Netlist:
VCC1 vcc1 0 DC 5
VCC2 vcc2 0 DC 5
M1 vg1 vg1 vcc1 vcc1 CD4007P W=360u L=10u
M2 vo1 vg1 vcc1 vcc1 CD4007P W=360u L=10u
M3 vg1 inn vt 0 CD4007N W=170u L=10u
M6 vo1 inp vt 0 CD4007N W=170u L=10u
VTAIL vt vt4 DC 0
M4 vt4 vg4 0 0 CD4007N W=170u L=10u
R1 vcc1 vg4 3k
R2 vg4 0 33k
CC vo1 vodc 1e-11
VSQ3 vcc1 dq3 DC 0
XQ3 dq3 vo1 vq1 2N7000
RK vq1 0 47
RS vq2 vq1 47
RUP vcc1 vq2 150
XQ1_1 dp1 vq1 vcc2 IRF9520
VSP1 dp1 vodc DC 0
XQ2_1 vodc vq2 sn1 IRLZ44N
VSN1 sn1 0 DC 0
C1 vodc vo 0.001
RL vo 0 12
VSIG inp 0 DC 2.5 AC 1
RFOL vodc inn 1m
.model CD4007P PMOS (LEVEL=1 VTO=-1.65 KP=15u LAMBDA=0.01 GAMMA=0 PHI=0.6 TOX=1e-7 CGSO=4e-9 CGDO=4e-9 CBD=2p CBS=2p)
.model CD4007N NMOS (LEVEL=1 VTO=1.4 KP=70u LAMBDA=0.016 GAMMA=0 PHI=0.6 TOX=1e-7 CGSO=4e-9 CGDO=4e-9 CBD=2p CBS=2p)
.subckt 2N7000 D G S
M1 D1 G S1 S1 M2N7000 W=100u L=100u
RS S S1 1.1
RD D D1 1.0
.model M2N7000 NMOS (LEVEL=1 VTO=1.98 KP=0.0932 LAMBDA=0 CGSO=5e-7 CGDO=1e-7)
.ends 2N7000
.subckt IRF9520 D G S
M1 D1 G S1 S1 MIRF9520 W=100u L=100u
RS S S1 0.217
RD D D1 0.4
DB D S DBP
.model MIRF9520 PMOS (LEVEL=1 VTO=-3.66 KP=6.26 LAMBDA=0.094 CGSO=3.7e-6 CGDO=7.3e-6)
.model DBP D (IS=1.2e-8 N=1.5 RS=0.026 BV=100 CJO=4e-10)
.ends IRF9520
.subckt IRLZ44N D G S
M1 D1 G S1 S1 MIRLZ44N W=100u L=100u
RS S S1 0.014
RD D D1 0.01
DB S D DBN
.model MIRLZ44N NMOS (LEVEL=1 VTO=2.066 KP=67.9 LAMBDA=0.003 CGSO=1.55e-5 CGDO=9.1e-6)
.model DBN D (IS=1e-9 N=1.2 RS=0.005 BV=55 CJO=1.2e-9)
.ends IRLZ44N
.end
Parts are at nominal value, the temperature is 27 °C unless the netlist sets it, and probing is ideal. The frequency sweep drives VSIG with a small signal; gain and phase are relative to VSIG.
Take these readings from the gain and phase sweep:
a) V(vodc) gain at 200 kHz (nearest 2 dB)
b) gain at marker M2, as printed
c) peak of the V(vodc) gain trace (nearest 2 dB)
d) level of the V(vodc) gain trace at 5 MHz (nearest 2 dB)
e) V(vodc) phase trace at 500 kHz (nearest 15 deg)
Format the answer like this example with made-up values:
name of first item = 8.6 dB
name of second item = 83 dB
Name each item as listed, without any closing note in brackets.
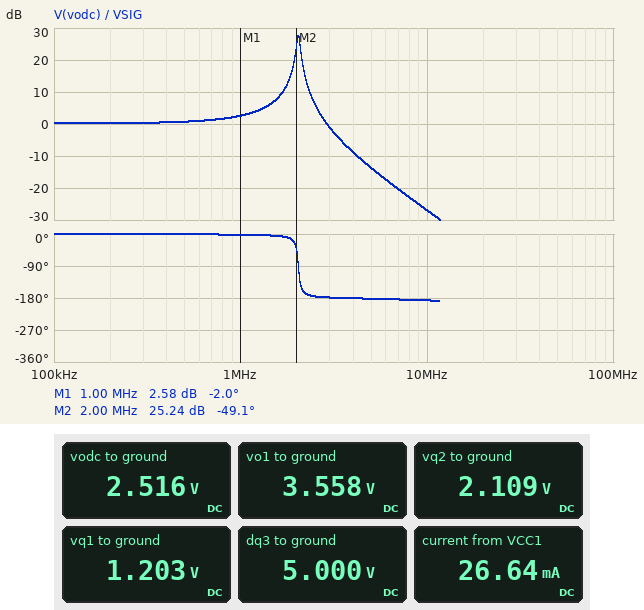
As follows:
V(vodc) gain at 200 kHz = 0 dB
gain at marker M2, as printed = 25.24 dB
peak of the V(vodc) gain trace = 28 dB
level of the V(vodc) gain trace at 5 MHz = -14 dB
V(vodc) phase trace at 500 kHz = 0 deg
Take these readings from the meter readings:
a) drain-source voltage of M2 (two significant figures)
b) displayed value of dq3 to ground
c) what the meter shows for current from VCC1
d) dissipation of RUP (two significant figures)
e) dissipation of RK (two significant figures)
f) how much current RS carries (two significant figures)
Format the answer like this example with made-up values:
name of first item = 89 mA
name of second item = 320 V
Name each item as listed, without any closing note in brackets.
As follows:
drain-source voltage of M2 = -1.4 V
displayed value of dq3 to ground = 5.000 V
what the meter shows for current from VCC1 = 26.64 mA
dissipation of RUP = 56 mW
dissipation of RK = 31 mW
how much current RS carries = 19 mA
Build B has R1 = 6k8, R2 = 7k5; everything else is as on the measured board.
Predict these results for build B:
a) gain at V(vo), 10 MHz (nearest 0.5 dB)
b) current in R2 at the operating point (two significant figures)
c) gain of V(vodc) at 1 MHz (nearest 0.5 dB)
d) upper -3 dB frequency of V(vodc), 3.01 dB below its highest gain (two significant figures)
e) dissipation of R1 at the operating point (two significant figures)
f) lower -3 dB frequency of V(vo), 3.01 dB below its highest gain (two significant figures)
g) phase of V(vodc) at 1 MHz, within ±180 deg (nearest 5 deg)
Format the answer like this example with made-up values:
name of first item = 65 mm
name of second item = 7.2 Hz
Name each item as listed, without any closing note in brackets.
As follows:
gain at V(vo), 10 MHz = -30.5 dB
current in R2 at the operating point = 350 µA
gain of V(vodc) at 1 MHz = 3.5 dB
upper -3 dB frequency of V(vodc), 3.01 dB below its highest gain = 1.8 MHz
dissipation of R1 at the operating point = 830 µW
lower -3 dB frequency of V(vo), 3.01 dB below its highest gain = 1.7 MHz
phase of V(vodc) at 1 MHz, within ±180 deg = -5 deg
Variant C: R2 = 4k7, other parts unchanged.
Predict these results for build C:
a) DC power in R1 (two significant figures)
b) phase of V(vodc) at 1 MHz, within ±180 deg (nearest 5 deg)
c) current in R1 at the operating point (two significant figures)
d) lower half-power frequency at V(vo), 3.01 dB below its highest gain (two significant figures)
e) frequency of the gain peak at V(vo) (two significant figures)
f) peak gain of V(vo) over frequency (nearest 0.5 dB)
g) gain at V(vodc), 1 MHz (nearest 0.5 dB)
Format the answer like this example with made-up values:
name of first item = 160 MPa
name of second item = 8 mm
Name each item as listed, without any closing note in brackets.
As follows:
DC power in R1 = 1.3 mW
phase of V(vodc) at 1 MHz, within ±180 deg = -5 deg
current in R1 at the operating point = 650 µA
lower half-power frequency at V(vo), 3.01 dB below its highest gain = 1.8 MHz
frequency of the gain peak at V(vo) = 1.9 MHz
peak gain of V(vo) over frequency = 25.5 dB
gain at V(vodc), 1 MHz = 3.0 dB
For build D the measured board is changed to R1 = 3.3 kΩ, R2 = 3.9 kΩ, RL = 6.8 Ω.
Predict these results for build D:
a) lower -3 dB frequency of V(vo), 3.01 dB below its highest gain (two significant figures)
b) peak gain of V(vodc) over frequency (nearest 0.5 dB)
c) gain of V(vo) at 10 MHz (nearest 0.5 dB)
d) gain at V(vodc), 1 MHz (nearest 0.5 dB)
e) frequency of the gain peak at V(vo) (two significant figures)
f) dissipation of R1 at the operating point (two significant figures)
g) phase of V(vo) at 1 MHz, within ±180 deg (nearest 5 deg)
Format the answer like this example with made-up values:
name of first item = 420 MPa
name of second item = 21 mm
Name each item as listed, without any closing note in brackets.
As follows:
lower -3 dB frequency of V(vo), 3.01 dB below its highest gain = 1.7 MHz
peak gain of V(vodc) over frequency = 21.5 dB
gain of V(vo) at 10 MHz = -30.5 dB
gain at V(vodc), 1 MHz = 3.5 dB
frequency of the gain peak at V(vo) = 1.8 MHz
dissipation of R1 at the operating point = 1.6 mW
phase of V(vo) at 1 MHz, within ±180 deg = -5 deg
